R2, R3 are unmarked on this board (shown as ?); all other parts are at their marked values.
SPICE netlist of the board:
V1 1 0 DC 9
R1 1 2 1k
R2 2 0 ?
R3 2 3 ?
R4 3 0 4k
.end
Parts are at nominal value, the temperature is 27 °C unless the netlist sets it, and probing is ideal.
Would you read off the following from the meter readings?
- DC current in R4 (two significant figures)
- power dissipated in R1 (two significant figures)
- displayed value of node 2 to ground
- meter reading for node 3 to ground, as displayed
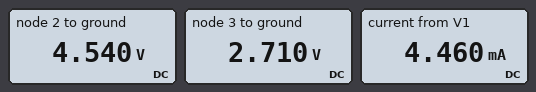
680 µA
20 mW
4.540 V
2.710 V
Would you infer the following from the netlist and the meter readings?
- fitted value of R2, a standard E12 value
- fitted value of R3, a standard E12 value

1.2 kΩ
2.7 kΩ
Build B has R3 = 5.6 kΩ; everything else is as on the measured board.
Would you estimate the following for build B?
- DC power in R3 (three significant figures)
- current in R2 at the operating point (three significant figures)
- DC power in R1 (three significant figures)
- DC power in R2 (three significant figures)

1.31 mW
3.87 mA
19.0 mW
18.0 mW
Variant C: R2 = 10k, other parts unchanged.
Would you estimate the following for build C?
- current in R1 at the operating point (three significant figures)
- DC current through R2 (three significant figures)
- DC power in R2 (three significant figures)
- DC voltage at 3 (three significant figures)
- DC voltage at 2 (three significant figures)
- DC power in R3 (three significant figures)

1.80 mA
720 µA
5.19 mW
4.30 V
7.20 V
3.12 mW
